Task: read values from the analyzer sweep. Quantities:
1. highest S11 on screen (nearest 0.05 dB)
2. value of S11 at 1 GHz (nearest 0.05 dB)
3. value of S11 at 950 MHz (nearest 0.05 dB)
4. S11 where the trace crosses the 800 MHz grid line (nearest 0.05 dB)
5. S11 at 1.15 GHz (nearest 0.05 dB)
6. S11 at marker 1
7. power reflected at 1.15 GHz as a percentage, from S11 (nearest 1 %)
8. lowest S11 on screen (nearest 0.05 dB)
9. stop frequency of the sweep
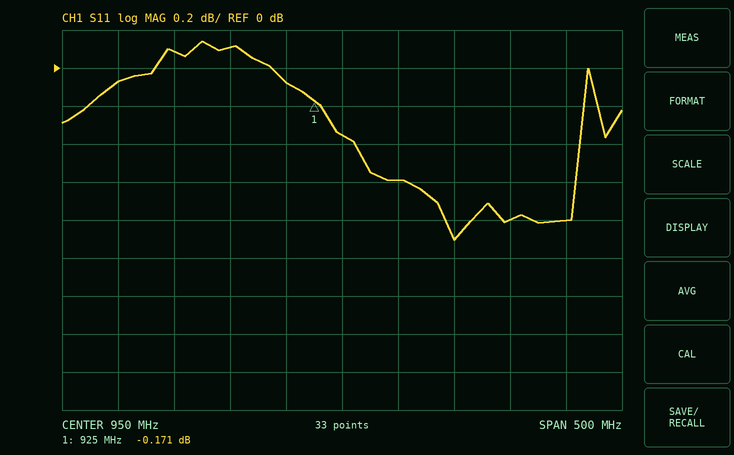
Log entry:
0.15 dB
-0.60 dB
-0.35 dB
0.10 dB
-0.80 dB
-0.171 dB
83 %
-0.90 dB
1.2 GHz
